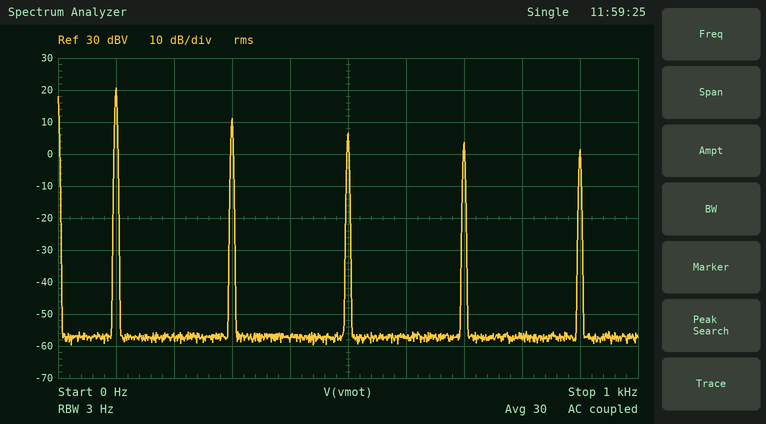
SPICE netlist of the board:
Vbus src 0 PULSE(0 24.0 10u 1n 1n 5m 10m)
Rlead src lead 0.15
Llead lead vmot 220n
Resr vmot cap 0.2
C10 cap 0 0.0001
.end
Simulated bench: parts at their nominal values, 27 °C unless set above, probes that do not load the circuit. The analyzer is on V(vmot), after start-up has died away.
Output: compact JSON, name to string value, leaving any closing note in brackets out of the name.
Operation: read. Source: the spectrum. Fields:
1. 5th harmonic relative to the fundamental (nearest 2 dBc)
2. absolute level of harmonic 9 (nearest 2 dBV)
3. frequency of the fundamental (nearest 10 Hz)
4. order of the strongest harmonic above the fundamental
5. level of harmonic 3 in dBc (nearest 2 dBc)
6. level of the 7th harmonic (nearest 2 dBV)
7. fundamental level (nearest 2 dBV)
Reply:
{"5th harmonic relative to the fundamental": "-14 dBc", "absolute level of harmonic 9": "2 dBV", "frequency of the fundamental": "100 Hz", "order of the strongest harmonic above the fundamental": "3", "level of harmonic 3 in dBc": "-10 dBc", "level of the 7th harmonic": "4 dBV", "fundamental level": "20 dBV"}
